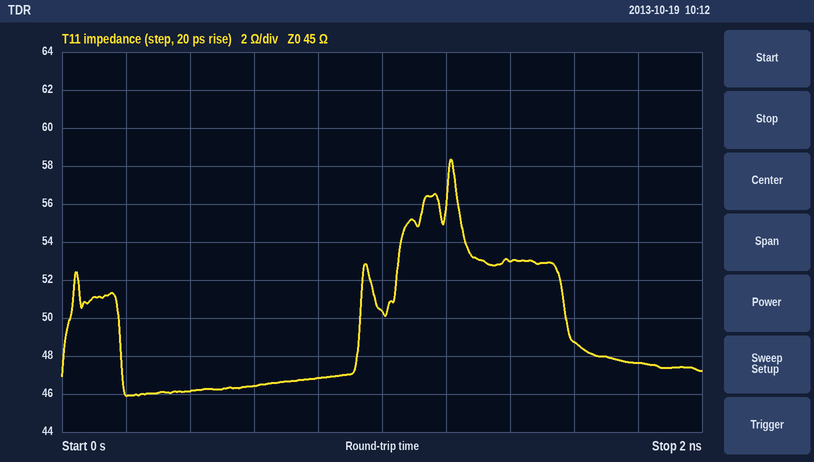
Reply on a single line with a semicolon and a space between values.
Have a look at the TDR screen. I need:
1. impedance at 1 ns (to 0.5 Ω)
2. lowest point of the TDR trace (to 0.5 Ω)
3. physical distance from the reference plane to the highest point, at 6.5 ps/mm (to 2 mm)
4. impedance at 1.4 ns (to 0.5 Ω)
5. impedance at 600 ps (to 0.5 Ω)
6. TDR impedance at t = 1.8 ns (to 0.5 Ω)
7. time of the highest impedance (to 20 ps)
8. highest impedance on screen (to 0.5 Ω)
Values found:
50.5 Ω; 46.0 Ω; 94 mm; 53.0 Ω; 46.5 Ω; 47.5 Ω; 1.22 ns; 58.5 Ω
